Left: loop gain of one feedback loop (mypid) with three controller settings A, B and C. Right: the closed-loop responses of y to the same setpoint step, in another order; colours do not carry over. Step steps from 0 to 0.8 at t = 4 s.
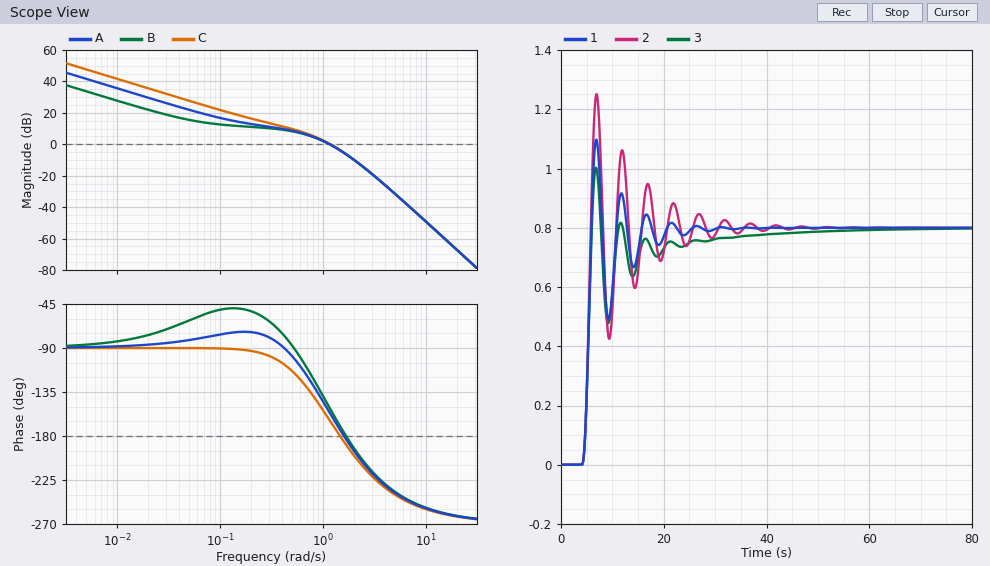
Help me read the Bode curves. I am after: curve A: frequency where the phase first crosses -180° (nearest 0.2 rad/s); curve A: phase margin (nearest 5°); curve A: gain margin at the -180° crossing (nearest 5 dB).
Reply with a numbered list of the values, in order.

1. 1.6 rad/s
2. 25°
3. 5 dB
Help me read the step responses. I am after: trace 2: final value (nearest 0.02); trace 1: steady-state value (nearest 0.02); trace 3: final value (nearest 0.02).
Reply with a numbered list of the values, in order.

1. 0.80
2. 0.80
3. 0.80
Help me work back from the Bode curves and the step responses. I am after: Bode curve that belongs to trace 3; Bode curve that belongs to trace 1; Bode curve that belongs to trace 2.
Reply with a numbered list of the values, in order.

1. B
2. A
3. C
